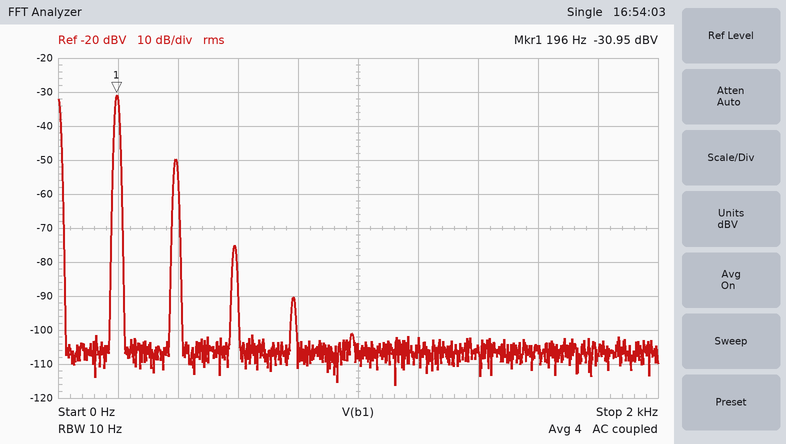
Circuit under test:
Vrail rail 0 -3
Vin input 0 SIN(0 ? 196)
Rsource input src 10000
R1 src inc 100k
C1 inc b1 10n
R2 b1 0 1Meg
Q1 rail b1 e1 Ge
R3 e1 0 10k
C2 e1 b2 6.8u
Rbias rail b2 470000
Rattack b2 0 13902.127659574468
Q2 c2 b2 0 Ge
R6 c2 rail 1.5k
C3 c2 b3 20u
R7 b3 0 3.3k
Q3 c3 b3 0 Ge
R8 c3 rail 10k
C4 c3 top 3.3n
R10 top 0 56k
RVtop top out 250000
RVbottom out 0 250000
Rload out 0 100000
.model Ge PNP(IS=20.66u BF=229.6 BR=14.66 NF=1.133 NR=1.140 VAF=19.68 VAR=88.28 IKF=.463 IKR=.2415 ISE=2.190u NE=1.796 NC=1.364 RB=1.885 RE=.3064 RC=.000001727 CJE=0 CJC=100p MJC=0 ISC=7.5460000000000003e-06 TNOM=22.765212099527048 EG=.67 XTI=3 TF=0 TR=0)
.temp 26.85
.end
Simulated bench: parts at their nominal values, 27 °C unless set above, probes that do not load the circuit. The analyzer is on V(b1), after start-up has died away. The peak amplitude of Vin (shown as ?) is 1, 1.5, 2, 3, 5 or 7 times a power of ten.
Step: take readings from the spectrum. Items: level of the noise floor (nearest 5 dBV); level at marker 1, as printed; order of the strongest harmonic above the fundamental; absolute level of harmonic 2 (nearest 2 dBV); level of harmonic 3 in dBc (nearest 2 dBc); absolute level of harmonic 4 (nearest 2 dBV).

-105 dBV
-30.95 dBV
2
-50 dBV
-44 dBc
-90 dBV
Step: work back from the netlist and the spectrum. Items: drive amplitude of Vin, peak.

150 mV
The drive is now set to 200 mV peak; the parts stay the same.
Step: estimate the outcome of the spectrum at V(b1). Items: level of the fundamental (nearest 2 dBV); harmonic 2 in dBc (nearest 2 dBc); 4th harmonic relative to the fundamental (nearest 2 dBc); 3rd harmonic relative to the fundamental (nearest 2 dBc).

-28 dBV
-16 dBc
-52 dBc
-40 dBc
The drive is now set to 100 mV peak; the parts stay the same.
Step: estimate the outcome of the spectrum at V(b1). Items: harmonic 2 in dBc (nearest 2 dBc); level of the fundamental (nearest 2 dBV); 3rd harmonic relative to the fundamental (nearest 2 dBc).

-22 dBc
-34 dBV
-50 dBc
